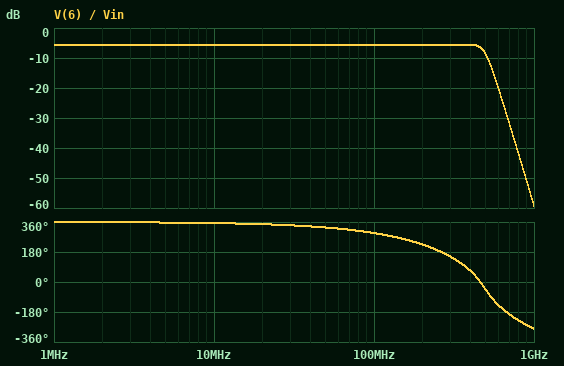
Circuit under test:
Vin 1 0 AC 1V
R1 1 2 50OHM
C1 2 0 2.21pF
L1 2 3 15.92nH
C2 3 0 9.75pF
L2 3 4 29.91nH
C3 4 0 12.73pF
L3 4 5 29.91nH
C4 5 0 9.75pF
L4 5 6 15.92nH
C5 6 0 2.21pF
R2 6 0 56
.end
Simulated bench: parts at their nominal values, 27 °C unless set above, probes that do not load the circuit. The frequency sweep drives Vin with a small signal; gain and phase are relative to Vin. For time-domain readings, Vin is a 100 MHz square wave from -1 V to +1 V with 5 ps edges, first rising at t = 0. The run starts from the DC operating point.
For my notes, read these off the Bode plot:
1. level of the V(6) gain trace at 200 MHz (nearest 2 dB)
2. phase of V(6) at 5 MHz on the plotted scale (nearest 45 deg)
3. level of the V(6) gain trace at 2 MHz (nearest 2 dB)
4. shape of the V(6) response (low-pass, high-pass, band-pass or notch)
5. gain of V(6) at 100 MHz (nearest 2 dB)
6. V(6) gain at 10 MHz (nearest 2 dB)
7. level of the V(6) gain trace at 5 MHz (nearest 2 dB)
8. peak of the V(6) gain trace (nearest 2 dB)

-6 dB
360 deg
-6 dB
low-pass
-6 dB
-6 dB
-6 dB
-6 dB
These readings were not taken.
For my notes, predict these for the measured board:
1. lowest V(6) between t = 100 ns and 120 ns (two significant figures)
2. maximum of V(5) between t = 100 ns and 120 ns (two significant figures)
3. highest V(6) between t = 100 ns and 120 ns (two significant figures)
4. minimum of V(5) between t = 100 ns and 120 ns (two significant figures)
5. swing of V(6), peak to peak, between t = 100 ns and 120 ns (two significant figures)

-720 mV
730 mV
720 mV
-730 mV
1.4 V
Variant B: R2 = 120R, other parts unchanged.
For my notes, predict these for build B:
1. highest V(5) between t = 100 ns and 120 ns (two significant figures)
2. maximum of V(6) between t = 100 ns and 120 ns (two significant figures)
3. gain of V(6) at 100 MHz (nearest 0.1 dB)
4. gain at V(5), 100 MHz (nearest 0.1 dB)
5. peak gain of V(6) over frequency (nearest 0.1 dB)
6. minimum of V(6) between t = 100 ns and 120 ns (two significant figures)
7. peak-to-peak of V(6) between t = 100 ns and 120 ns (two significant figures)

890 mV
950 mV
-3.0 dB
-3.1 dB
-2.6 dB
-950 mV
1.9 V
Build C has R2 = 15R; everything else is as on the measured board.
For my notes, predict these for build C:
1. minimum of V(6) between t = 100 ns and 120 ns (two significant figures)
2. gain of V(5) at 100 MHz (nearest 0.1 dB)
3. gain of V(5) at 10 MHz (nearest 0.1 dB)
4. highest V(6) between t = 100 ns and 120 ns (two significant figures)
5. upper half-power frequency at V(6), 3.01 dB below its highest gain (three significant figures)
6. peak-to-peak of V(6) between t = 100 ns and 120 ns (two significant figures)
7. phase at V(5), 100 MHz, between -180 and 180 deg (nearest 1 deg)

-310 mV
-11.2 dB
-12.7 dB
310 mV
553 MHz
630 mV
-32 deg
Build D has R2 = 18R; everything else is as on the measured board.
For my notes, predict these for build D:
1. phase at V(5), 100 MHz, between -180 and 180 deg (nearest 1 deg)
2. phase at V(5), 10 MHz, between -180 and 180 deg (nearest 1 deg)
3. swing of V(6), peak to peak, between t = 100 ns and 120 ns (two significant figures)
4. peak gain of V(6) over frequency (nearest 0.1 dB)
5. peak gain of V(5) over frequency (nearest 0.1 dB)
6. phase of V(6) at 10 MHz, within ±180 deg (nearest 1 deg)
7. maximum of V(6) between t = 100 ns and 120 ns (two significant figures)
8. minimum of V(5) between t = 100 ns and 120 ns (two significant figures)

-37 deg
-3 deg
720 mV
-11.5 dB
-3.3 dB
-7 deg
360 mV
-650 mV
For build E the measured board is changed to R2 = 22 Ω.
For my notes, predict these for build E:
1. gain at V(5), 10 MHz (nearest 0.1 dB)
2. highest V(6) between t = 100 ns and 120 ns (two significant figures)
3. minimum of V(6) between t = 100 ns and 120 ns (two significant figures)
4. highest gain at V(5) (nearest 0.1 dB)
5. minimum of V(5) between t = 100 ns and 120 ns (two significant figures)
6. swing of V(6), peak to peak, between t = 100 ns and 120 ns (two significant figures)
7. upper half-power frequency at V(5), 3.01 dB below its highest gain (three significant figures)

-10.3 dB
420 mV
-420 mV
-4.2 dB
-650 mV
830 mV
555 MHz
